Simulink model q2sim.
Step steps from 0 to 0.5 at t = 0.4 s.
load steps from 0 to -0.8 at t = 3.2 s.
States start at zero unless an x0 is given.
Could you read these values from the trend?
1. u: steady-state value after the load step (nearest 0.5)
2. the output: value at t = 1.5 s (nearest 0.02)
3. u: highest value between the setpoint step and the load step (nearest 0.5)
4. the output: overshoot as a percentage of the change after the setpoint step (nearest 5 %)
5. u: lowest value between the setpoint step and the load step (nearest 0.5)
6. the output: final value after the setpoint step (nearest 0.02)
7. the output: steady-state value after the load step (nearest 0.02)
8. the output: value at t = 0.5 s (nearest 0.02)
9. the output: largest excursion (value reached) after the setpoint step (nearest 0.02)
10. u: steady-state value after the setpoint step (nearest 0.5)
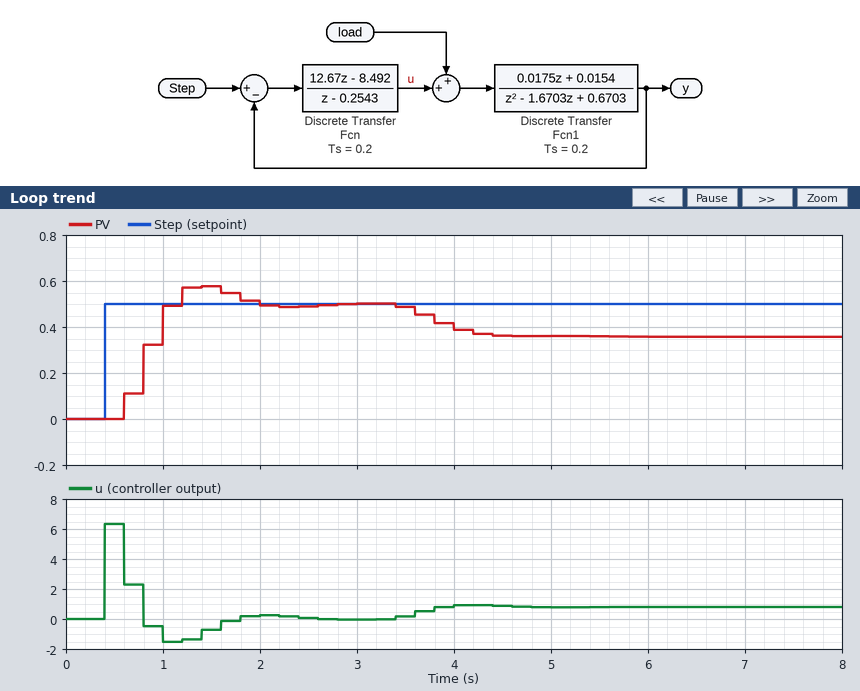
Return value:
1.0
0.58
6.5
15 %
-1.5
0.50
0.36
0.00
0.58
0.0
